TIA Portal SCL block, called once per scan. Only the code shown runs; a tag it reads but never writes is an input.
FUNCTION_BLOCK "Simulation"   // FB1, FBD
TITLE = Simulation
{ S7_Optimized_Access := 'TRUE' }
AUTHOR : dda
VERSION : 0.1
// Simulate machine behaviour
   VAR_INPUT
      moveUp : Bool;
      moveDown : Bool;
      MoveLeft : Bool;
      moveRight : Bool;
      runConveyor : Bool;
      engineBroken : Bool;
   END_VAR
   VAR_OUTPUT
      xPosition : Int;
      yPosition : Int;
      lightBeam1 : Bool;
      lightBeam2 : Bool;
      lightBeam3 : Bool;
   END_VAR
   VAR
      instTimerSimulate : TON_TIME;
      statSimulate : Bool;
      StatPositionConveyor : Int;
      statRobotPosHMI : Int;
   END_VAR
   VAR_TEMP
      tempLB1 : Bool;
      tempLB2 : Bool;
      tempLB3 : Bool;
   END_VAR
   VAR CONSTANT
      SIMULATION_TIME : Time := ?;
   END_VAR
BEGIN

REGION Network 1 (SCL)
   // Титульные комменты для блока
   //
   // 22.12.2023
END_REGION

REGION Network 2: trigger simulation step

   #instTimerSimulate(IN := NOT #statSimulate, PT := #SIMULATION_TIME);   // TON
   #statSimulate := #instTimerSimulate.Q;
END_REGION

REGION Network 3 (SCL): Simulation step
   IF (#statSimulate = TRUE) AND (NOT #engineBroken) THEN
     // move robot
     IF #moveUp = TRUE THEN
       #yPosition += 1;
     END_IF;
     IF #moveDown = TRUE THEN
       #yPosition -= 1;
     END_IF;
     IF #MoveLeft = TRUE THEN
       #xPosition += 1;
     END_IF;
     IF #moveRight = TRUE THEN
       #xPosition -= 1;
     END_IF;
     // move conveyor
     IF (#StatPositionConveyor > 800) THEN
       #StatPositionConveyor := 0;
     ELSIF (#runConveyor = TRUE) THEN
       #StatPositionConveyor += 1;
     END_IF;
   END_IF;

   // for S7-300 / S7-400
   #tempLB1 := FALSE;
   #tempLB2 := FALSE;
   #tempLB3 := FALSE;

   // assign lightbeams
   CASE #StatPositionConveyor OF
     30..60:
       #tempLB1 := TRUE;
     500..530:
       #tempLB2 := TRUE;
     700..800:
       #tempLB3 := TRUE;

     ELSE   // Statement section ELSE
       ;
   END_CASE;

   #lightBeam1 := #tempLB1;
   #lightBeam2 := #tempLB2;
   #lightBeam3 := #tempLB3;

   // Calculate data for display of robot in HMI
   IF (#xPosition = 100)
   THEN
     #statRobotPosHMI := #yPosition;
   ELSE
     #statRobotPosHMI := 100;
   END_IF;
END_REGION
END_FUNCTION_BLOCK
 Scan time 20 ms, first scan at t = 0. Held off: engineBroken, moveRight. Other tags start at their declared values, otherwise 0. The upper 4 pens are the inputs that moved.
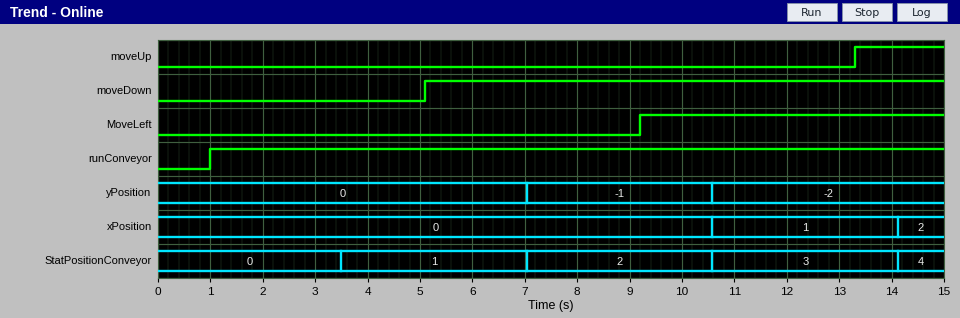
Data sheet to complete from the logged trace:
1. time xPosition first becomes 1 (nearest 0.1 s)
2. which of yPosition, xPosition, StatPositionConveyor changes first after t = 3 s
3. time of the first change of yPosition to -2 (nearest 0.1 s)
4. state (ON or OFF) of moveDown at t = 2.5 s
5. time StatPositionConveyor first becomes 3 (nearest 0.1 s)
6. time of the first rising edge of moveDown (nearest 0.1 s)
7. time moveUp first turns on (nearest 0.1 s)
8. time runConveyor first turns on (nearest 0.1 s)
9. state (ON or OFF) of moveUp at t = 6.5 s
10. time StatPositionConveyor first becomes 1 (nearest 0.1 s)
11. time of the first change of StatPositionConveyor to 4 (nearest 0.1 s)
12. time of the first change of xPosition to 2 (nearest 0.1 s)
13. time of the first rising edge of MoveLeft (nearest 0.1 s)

10.6 s
StatPositionConveyor
10.6 s
OFF
10.6 s
5.1 s
13.3 s
1.0 s
OFF
3.5 s
14.1 s
14.1 s
9.2 s
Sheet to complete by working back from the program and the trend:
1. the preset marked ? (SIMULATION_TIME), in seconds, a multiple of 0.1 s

3.5 s
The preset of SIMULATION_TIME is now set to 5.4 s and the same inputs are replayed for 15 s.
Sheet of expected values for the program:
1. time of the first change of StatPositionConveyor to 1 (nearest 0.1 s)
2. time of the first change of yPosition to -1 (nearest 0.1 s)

5.4 s
5.4 s
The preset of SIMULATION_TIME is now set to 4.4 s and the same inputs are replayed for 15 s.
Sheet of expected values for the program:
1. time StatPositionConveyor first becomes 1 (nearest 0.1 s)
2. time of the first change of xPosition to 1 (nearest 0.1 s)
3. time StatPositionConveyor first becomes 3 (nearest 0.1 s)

4.4 s
13.3 s
13.3 s
